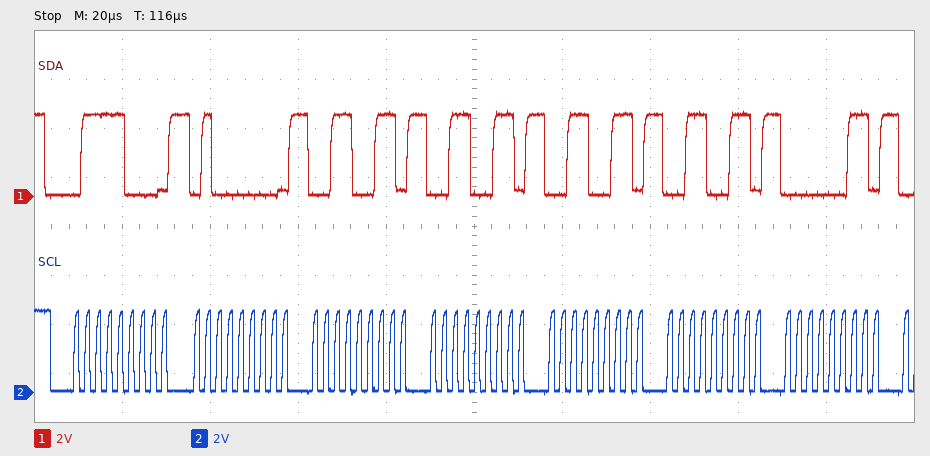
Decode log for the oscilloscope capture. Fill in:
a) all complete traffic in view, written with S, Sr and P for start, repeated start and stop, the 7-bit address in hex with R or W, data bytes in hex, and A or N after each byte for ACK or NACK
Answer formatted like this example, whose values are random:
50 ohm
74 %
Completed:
S 3CW A 40 A 33 A 33 A 33 A 33 A 03 A
